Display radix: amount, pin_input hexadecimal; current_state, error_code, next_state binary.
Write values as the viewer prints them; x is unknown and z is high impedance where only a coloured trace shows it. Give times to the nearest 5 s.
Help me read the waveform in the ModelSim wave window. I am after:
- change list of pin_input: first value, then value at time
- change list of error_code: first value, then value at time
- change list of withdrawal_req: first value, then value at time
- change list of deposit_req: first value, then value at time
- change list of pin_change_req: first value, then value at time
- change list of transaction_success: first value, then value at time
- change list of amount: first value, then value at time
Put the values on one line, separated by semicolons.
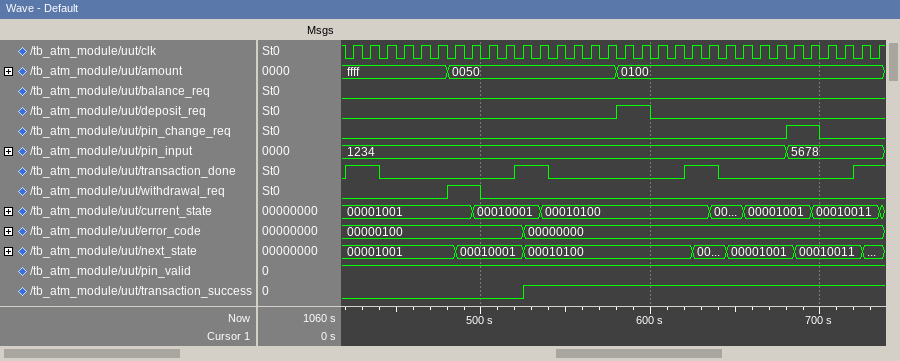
1234, 5678 at 680 s; 00000100, 00000000 at 525 s; 0, 1 at 480 s, 0 at 500 s; 0, 1 at 580 s, 0 at 600 s; 0, 1 at 680 s, 0 at 700 s; 0, 1 at 525 s; ffff, 0050 at 480 s, 0100 at 580 s
